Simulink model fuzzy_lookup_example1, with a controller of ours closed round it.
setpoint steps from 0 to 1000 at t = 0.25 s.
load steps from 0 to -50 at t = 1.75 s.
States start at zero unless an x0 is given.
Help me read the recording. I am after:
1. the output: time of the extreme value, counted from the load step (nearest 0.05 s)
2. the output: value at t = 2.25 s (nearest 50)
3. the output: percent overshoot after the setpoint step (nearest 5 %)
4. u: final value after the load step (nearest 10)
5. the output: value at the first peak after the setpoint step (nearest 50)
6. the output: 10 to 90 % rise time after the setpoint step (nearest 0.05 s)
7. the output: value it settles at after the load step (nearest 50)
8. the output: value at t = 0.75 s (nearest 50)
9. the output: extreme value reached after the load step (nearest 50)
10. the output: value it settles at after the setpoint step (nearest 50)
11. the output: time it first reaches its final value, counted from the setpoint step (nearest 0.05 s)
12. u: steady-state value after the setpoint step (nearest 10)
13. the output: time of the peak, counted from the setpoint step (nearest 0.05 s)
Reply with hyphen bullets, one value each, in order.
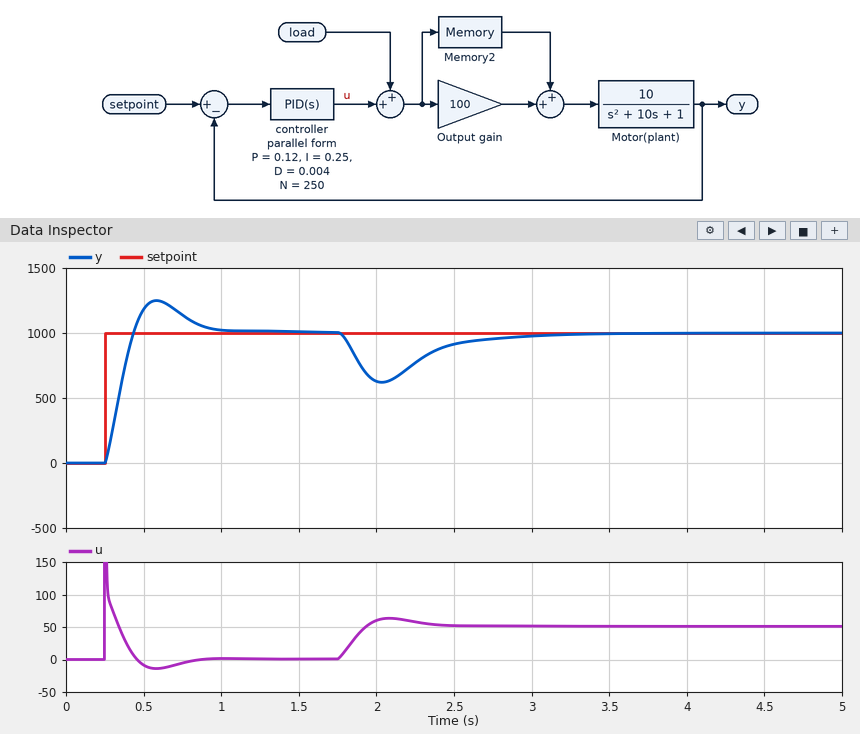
- 0.30 s
- 750
- 25 %
- 50
- 1250
- 0.15 s
- 1000
- 1150
- 600
- 1000
- 0.20 s
- 0
- 0.35 s
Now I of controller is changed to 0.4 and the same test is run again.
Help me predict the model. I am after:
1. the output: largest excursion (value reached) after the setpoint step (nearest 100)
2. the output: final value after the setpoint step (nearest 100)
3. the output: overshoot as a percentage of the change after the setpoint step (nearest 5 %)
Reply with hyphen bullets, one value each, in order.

- 1300
- 1000
- 35 %
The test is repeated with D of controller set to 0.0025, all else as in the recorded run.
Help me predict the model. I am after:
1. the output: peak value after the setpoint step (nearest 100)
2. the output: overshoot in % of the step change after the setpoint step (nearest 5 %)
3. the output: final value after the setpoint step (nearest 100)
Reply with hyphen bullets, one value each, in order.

- 1300
- 30 %
- 1000
